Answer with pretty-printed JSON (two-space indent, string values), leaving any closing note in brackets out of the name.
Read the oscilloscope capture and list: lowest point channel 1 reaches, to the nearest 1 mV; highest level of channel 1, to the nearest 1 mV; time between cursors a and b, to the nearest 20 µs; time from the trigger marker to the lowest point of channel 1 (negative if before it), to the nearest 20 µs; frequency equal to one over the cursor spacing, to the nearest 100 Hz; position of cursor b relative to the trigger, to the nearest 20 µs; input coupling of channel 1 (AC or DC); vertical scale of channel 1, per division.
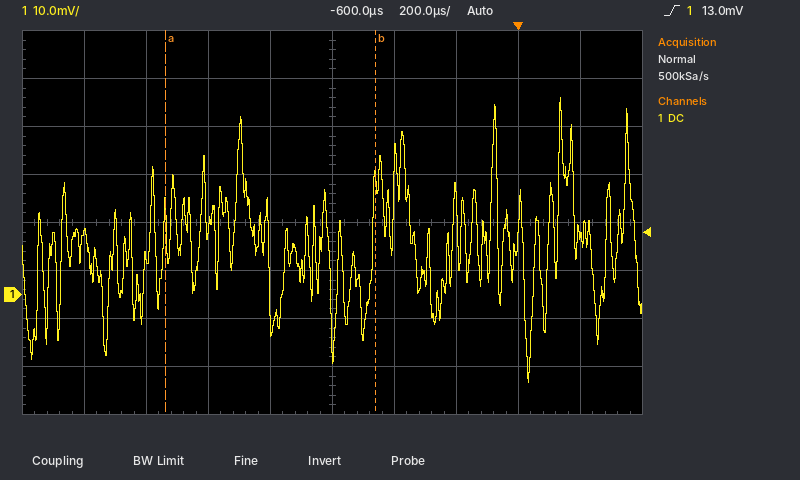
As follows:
{
  "lowest point channel 1 reaches, to the nearest 1 mV": "-18 mV",
  "highest level of channel 1, to the nearest 1 mV": "41 mV",
  "time between cursors a and b, to the nearest 20 µs": "680 µs",
  "time from the trigger marker to the lowest point of channel 1 (negative if before it), to the nearest 20 µs": "+40 µs",
  "frequency equal to one over the cursor spacing, to the nearest 100 Hz": "1.5 kHz",
  "position of cursor b relative to the trigger, to the nearest 20 µs": "-460 µs",
  "input coupling of channel 1": "DC",
  "vertical scale of channel 1, per division": "10 mV"
}
